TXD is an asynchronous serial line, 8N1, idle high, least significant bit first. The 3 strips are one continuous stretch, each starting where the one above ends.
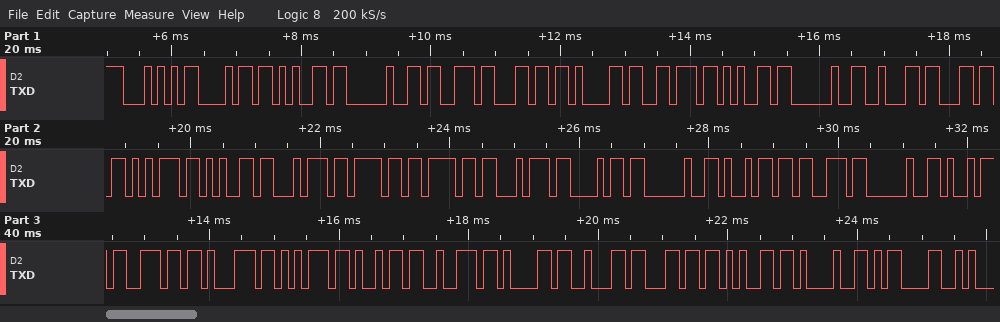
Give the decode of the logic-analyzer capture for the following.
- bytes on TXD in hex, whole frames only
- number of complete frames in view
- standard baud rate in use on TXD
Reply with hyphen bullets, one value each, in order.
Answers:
- 54 68 65 20 73 6C 61 76 65 20 62 6C 75 65 74 6F 6F 74 68 20 69 73 20 69 6E 71 75 69 72 61 62 6C 65 21 0D
- 35
- 9600 baud
